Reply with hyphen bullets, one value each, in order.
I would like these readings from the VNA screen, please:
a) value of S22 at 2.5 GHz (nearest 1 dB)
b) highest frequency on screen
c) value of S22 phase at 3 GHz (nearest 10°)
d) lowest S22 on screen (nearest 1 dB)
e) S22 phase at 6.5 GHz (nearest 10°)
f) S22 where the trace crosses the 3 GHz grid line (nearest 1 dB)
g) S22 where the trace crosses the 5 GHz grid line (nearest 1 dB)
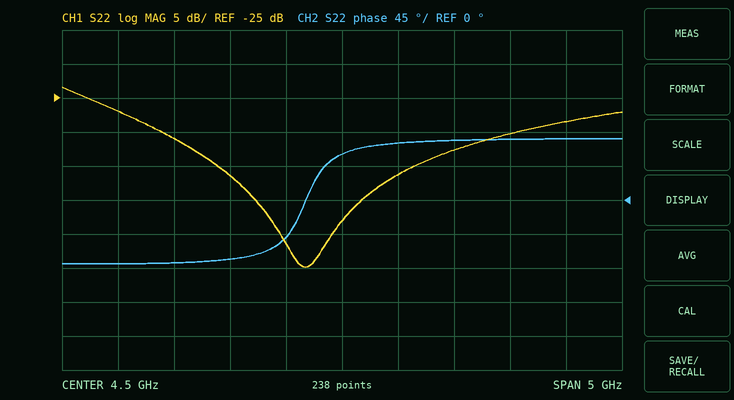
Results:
- -27 dB
- 7 GHz
- -80°
- -50 dB
- 80°
- -31 dB
- -36 dB
